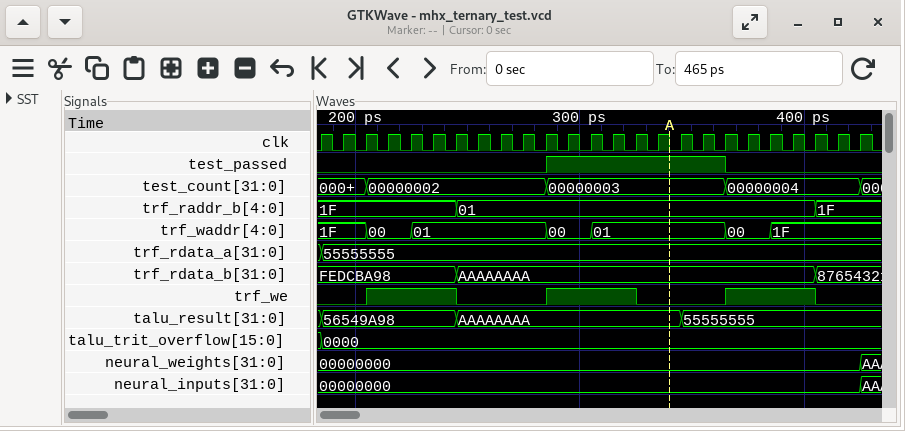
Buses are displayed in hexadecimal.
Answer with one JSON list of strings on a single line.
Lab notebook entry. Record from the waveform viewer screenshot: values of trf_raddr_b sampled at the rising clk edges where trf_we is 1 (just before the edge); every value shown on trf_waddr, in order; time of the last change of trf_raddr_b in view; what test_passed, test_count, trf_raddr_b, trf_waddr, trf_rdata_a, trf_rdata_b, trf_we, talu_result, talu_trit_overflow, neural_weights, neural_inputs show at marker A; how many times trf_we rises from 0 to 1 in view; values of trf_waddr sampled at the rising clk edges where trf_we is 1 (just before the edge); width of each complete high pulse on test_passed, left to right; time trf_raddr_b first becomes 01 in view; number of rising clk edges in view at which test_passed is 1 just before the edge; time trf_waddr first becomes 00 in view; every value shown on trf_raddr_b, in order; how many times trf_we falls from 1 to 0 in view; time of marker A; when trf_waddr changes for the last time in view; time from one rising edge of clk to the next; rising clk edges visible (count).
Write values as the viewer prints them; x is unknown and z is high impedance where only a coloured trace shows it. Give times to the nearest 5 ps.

["1F, 1F, 1F, 1F, 01, 01, 01, 01, 01, 01, 01, 01", "1F, 00, 01, 00, 01, 00, 1F", "405 ps", "test_passed=1, test_count=00000003, trf_raddr_b=01, trf_waddr=01, trf_rdata_a=55555555, trf_rdata_b=AAAAAAAA, trf_we=0, talu_result=AAAAAAAA, talu_trit_overflow=0000, neural_weights=00000000, neural_inputs=00000000", "3", "00, 00, 01, 01, 00, 00, 01, 01, 00, 00, 1F, 1F", "80 ps", "245 ps", "8", "205 ps", "1F, 01, 1F", "3", "340 ps", "385 ps", "10 ps", "25"]
